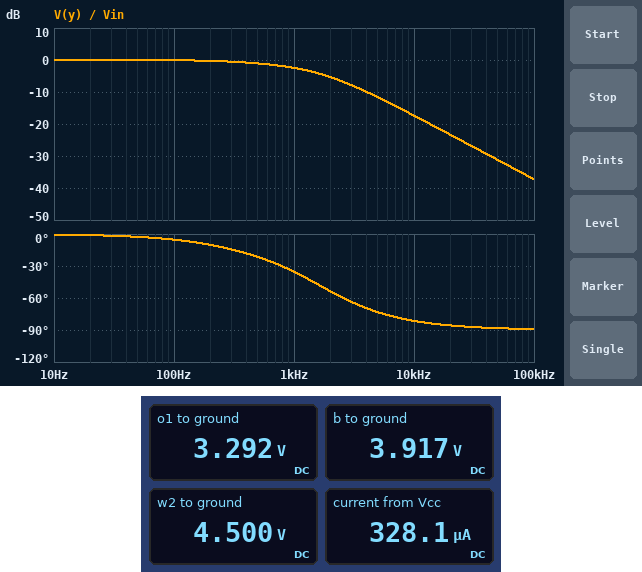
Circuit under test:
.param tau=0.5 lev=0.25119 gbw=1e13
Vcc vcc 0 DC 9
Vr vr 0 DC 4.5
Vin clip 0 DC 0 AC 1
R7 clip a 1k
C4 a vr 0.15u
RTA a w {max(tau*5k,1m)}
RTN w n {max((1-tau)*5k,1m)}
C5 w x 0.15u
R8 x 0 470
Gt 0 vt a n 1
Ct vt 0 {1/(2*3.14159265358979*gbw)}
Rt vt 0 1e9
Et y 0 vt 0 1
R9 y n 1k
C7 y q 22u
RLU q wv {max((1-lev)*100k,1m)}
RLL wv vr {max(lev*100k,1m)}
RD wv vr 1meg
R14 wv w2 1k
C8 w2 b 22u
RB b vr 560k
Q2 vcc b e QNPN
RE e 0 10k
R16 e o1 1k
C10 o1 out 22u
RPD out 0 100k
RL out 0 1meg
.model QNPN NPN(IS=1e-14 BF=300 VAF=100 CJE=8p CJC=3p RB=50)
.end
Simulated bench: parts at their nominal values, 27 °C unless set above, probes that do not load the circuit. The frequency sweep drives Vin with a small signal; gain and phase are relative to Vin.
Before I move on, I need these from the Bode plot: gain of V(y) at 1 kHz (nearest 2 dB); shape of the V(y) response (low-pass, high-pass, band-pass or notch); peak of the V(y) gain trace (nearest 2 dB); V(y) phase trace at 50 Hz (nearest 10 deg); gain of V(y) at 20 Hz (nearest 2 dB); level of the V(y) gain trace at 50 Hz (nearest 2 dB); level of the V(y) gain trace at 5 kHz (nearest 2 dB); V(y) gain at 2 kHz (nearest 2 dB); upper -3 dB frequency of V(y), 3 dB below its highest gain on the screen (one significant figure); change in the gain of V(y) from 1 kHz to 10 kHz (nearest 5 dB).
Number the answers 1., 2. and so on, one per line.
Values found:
1. -2 dB
2. low-pass
3. 0 dB
4. 0 deg
5. 0 dB
6. 0 dB
7. -12 dB
8. -6 dB
9. 1 kHz
10. -15 dB
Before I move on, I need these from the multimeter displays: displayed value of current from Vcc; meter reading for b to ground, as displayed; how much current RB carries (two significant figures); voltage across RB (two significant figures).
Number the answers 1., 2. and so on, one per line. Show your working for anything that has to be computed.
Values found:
1. 328.1 µA
2. 3.917 V
3. (4.5 V - 3.917 V) / 560 kΩ = 1.0 µA
4. 4.5 V - 3.917 V = 580 mV
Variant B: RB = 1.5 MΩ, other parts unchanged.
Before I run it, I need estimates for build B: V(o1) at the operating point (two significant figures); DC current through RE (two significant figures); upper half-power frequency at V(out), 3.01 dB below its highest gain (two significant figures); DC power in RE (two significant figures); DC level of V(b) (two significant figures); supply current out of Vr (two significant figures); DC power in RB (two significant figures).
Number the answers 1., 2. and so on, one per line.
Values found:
1. 2.6 V
2. 260 µA
3. 1.2 kHz
4. 700 µW
5. 3.3 V
6. 830 nA
7. 1.0 µW
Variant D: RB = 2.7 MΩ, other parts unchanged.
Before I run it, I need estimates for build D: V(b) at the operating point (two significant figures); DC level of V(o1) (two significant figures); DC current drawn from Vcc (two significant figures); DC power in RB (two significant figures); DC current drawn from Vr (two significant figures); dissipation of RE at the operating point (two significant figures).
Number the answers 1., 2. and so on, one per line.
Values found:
1. 2.7 V
2. 2.1 V
3. 210 µA
4. 1.2 µW
5. 660 nA
6. 440 µW
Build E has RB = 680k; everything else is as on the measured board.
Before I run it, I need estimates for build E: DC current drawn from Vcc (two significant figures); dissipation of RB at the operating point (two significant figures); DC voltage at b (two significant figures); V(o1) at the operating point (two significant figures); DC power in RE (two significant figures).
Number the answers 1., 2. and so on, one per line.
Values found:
1. 320 µA
2. 690 nW
3. 3.8 V
4. 3.2 V
5. 1.0 mW
